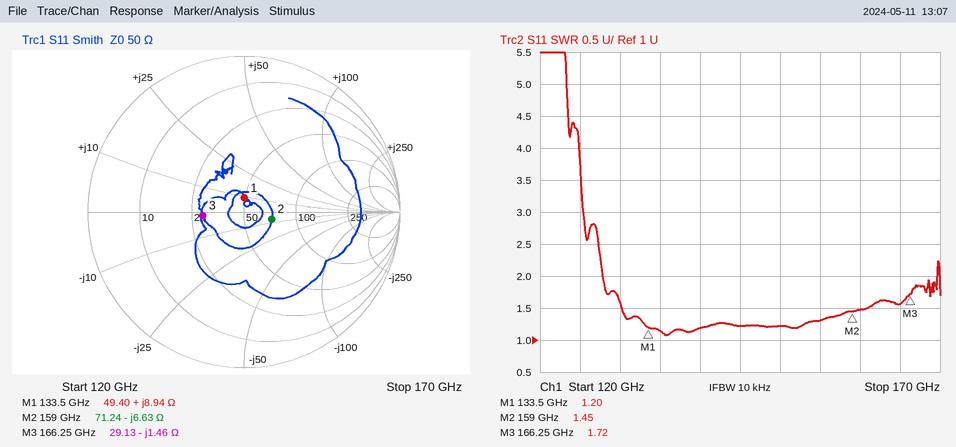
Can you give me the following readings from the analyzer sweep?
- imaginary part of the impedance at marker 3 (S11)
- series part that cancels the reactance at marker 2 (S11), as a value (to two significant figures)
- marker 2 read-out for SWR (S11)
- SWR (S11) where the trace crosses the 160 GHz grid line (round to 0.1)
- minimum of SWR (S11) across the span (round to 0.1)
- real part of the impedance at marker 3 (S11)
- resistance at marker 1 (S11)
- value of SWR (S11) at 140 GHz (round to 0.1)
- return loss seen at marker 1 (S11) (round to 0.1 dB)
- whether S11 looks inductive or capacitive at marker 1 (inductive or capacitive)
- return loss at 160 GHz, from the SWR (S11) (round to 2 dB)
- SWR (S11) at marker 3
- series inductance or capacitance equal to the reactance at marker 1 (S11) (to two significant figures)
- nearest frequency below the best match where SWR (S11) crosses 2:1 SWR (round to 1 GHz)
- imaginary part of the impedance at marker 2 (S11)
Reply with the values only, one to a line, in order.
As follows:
-1.46 Ω
6.6 pH
1.45
1.5
1.1
29.13 Ω
49.40 Ω
1.2
20.9 dB
inductive
14 dB
1.72
11 pH
128 GHz
-6.63 Ω
